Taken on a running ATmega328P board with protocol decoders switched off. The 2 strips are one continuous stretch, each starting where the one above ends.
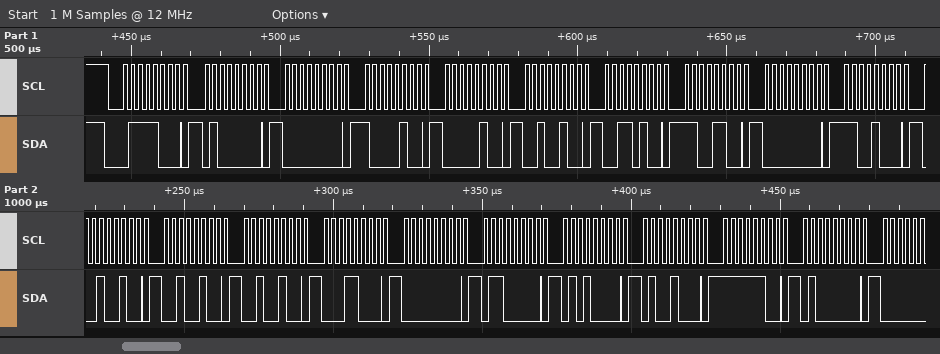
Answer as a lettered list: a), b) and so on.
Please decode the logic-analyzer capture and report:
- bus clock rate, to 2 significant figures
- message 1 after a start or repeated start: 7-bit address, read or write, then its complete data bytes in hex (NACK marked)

a) 400 kHz
b) 0x3C write: 40 00 84 04 24 34 CC 00 C8 24 24 24 18 00 60 50 48 FC 40
